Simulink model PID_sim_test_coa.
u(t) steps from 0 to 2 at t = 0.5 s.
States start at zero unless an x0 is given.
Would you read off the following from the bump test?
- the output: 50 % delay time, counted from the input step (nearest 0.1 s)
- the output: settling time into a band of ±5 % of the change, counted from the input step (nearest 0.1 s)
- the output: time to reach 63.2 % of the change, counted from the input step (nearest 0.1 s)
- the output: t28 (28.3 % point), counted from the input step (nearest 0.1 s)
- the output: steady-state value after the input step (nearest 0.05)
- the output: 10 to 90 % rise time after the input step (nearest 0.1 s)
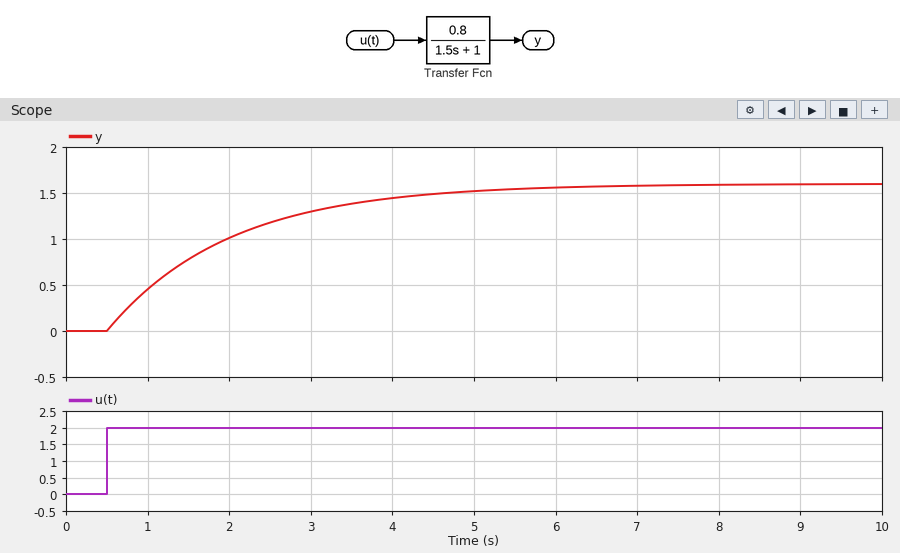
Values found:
1.0 s
4.5 s
1.5 s
0.5 s
1.60
3.3 s
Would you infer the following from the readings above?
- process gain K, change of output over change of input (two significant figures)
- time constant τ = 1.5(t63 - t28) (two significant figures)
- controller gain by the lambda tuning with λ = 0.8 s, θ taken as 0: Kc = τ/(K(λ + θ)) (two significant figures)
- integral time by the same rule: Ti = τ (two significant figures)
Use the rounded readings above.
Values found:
0.80
1.5 s
2.3
1.5 s
